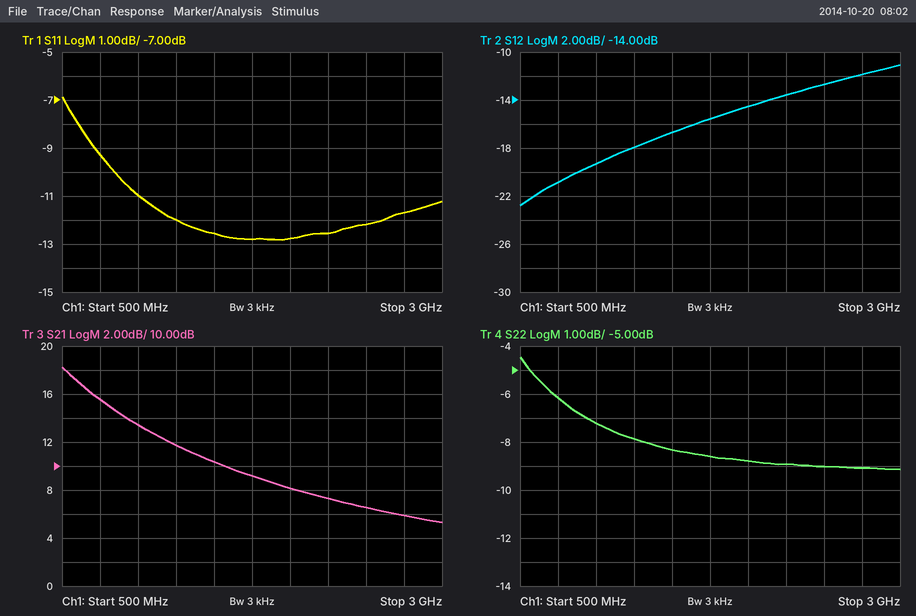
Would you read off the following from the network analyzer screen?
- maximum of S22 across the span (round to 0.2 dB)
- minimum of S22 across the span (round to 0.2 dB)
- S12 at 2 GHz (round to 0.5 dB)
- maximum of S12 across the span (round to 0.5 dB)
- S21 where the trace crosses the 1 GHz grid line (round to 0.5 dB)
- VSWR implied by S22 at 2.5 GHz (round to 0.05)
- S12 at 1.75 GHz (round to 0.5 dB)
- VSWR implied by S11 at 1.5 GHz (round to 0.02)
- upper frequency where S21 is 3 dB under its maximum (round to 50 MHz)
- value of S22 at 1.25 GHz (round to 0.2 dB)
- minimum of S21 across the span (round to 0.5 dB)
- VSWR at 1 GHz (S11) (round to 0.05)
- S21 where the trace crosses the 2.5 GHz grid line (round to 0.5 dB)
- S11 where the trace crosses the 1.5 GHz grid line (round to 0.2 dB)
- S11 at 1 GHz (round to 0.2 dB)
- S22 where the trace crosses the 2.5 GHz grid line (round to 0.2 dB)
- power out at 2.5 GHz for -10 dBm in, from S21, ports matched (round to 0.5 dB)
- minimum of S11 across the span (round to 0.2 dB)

-4.4 dB
-9.2 dB
-14.5 dB
-11.0 dB
13.5 dB
2.10
-15.5 dB
1.62
800 MHz
-7.8 dB
5.5 dB
1.80
6.5 dB
-12.6 dB
-11.0 dB
-9.0 dB
-3.5 dBm
-12.8 dB
